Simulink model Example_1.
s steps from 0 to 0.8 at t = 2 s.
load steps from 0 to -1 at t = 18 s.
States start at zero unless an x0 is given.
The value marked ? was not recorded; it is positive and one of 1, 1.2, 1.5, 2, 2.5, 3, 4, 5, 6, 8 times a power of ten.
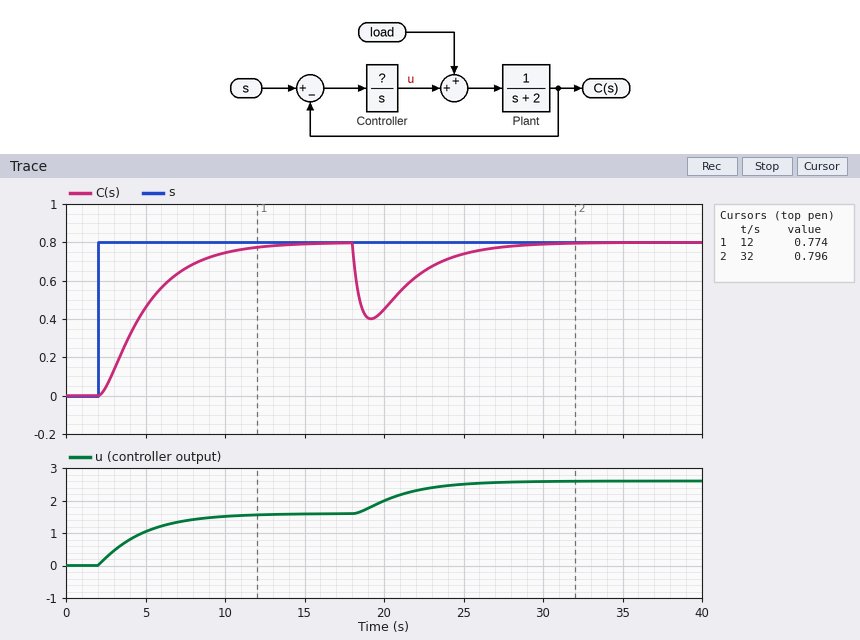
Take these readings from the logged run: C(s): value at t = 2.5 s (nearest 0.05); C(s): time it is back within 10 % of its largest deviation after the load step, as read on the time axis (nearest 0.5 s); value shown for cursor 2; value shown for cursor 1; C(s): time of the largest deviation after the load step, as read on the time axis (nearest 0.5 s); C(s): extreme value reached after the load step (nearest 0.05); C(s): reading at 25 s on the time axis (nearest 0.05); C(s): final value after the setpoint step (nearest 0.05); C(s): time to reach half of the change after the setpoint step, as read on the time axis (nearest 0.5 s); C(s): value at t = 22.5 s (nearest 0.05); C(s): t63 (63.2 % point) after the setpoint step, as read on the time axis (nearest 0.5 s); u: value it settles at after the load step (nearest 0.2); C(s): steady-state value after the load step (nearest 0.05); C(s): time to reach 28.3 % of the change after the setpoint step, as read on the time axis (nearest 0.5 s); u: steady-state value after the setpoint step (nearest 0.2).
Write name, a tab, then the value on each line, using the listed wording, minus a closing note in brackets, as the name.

C(s): value at t = 2.5 s	0.05
C(s): time it is back within 10 % of its largest deviation after the load step, as read on the time axis	26.0 s
value shown for cursor 2	0.796
value shown for cursor 1	0.774
C(s): time of the largest deviation after the load step, as read on the time axis	19.0 s
C(s): extreme value reached after the load step	0.40
C(s): reading at 25 s on the time axis	0.75
C(s): final value after the setpoint step	0.80
C(s): time to reach half of the change after the setpoint step, as read on the time axis	4.5 s
C(s): value at t = 22.5 s	0.65
C(s): t63 (63.2 % point) after the setpoint step, as read on the time axis	5.5 s
u: value it settles at after the load step	2.6
C(s): steady-state value after the load step	0.80
C(s): time to reach 28.3 % of the change after the setpoint step, as read on the time axis	3.5 s
u: steady-state value after the setpoint step	1.6
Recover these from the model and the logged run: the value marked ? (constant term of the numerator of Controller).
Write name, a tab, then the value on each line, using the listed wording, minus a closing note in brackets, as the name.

the value marked ?	0.6
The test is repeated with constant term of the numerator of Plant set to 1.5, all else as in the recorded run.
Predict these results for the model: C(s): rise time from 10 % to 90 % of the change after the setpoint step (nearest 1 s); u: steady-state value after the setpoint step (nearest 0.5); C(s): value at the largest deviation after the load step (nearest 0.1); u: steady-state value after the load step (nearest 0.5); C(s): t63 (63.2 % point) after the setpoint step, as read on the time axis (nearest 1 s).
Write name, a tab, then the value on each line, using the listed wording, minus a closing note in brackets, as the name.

C(s): rise time from 10 % to 90 % of the change after the setpoint step	4 s
u: steady-state value after the setpoint step	1.0
C(s): value at the largest deviation after the load step	0.2
u: steady-state value after the load step	2.0
C(s): t63 (63.2 % point) after the setpoint step, as read on the time axis	4 s
